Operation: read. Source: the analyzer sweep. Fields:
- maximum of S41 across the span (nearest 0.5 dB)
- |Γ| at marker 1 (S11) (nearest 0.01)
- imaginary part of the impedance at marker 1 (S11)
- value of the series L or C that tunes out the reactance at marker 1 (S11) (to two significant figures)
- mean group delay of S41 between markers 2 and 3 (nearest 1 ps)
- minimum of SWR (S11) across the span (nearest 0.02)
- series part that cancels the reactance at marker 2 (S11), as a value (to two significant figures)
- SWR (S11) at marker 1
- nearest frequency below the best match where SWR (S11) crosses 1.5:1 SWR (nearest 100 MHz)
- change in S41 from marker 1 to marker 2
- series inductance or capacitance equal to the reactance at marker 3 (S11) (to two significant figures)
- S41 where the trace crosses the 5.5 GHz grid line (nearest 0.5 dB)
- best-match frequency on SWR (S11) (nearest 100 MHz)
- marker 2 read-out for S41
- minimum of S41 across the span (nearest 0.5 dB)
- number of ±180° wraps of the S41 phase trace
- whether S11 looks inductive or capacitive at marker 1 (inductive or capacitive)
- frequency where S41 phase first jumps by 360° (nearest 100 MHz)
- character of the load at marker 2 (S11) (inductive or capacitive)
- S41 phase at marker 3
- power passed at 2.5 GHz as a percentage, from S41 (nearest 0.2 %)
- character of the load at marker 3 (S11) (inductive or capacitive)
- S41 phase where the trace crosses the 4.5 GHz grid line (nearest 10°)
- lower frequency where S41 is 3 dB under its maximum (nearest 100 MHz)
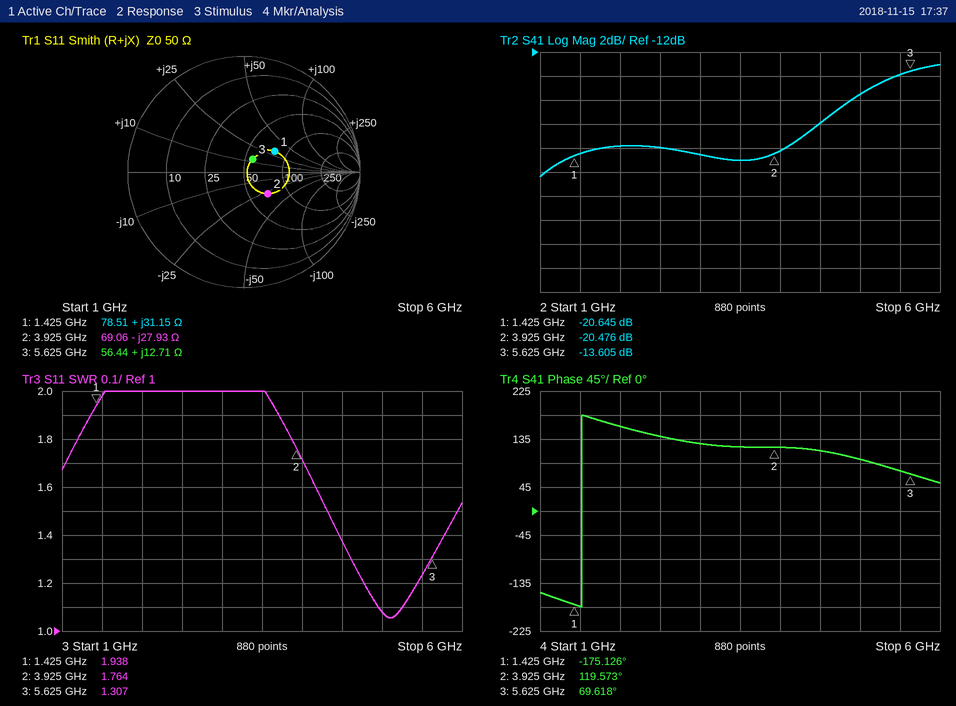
-13.0 dB
0.32
+31.15 Ω
3.6 pF
82 ps
1.06
1.1 nH
1.938
4.3 GHz
0.169 dB
360 pH
-14.0 dB
5.1 GHz
-20.476 dB
-22.5 dB
1
inductive
1.5 GHz
capacitive
69.618°
1.0 %
inductive
110°
4.9 GHz
